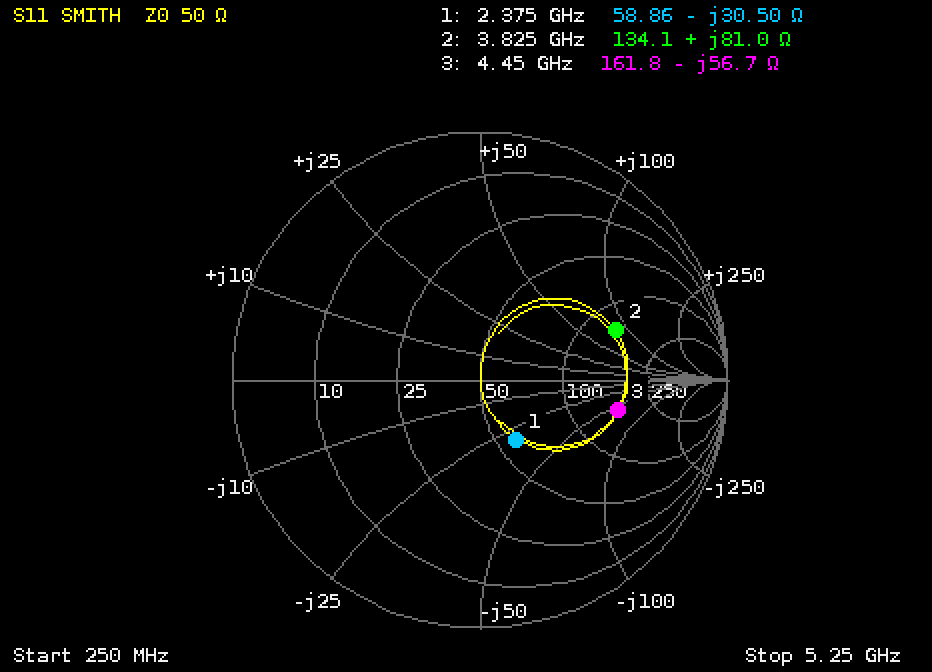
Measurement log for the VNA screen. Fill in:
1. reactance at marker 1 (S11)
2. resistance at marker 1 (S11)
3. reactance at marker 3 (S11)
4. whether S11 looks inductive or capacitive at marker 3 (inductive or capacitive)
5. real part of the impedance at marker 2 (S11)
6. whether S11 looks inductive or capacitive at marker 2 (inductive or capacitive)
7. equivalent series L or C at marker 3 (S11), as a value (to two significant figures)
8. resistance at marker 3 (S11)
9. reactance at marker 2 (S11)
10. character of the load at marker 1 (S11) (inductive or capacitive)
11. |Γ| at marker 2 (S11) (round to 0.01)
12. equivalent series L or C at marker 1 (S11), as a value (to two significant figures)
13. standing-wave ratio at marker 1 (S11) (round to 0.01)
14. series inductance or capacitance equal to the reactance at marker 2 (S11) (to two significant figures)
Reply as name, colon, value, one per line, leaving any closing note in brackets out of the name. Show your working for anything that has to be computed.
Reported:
reactance at marker 1: -30.50 Ω
resistance at marker 1: 58.86 Ω
reactance at marker 3: -56.7 Ω
whether S11 looks inductive or capacitive at marker 3: capacitive
real part of the impedance at marker 2: 134.1 Ω
whether S11 looks inductive or capacitive at marker 2: inductive
equivalent series L or C at marker 3 (S11), as a value: C = 1/(2π × 4.45 GHz × 56.7 Ω) ≈ 631 fF, so 630 fF to two significant figures
resistance at marker 3: 161.8 Ω
reactance at marker 2: +81.0 Ω
character of the load at marker 1 (S11): capacitive
|Γ| at marker 2 (S11): 0.58
equivalent series L or C at marker 1 (S11), as a value: C = 1/(2π × 2.375 GHz × 30.5 Ω) ≈ 2.2 pF
standing-wave ratio at marker 1 (S11): 1.78
series inductance or capacitance equal to the reactance at marker 2 (S11): L = 81 Ω/(2π × 3.825 GHz) ≈ 3.4 nH
